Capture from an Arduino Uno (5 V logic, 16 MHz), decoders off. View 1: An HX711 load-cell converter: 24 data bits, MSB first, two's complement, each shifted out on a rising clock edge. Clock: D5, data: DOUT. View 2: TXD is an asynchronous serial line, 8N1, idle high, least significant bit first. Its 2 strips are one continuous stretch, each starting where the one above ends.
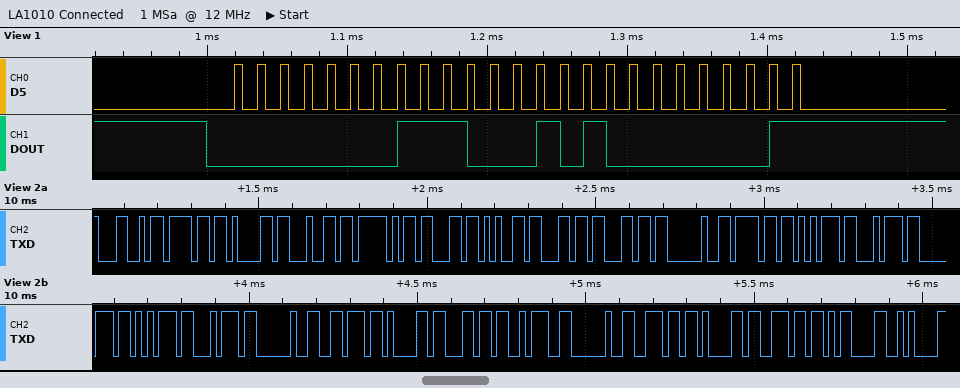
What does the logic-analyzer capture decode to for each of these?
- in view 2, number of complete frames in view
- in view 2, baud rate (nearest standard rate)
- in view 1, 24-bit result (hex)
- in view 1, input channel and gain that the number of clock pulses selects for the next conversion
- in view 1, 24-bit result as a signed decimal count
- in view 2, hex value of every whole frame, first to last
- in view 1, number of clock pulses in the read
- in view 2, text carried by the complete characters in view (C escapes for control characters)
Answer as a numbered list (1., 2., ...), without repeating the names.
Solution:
1. 27
2. 57600 baud
3. 0x01C501
4. channel A, gain 128
5. 115969
6. 4C 6F 61 64 5F 63 65 6C 6C 20 6F 75 74 70 75 74 20 76 61 6C 3A 20 6E 61 6E 0D 0A
7. 25
8. "Load_cell output val: nan\r\n"
